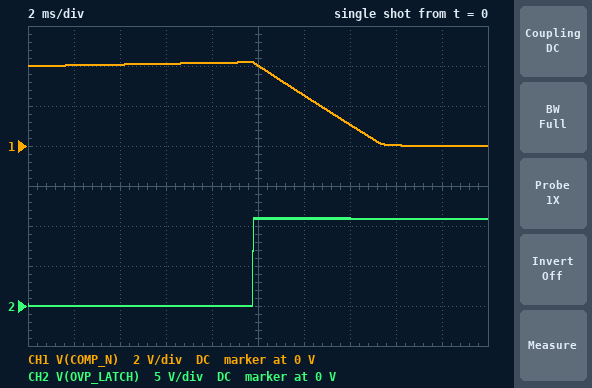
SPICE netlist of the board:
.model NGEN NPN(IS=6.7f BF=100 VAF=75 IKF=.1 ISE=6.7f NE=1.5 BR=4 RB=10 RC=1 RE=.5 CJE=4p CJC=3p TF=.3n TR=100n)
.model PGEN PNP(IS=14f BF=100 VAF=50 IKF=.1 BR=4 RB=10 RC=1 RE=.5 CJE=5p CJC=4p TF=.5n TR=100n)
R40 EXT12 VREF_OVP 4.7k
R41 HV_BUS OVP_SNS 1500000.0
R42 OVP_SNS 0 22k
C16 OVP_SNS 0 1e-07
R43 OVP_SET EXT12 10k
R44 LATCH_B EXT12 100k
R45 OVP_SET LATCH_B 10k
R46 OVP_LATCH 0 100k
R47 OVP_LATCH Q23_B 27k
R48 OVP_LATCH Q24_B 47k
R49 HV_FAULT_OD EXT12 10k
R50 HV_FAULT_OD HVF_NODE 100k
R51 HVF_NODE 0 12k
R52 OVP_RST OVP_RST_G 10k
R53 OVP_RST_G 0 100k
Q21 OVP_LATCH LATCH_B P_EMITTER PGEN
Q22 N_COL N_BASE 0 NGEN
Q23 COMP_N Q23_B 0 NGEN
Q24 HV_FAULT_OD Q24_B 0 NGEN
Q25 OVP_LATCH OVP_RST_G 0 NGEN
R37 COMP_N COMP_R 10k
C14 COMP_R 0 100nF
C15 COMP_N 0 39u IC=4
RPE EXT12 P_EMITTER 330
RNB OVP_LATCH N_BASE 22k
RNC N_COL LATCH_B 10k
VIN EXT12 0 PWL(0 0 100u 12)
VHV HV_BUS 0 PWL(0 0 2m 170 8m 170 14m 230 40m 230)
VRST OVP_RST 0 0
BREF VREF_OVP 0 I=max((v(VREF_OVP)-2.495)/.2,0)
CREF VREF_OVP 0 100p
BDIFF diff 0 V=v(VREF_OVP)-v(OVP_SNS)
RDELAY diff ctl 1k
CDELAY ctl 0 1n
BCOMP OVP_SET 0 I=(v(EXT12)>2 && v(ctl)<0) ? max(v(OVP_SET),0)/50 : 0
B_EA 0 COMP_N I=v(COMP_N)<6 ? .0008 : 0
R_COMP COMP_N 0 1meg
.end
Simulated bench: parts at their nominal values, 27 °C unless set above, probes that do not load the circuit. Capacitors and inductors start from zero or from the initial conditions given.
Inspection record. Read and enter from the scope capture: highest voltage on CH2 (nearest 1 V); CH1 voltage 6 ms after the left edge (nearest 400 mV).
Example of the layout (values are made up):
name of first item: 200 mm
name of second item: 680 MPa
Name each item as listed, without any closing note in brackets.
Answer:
highest voltage on CH2: 11 V
CH1 voltage 6 ms after the left edge: 4.0 V
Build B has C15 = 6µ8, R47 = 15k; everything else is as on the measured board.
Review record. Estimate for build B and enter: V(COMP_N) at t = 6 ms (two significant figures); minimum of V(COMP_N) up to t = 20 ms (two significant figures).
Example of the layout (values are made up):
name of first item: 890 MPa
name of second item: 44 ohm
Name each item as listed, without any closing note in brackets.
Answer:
V(COMP_N) at t = 6 ms: 4.6 V
minimum of V(COMP_N) up to t = 20 ms: 14 mV
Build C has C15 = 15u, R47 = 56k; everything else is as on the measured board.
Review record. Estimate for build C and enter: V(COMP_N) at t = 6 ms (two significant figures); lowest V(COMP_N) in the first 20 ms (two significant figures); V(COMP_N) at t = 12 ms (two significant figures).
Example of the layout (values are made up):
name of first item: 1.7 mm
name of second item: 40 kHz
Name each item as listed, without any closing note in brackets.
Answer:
V(COMP_N) at t = 6 ms: 4.3 V
lowest V(COMP_N) in the first 20 ms: 25 mV
V(COMP_N) at t = 12 ms: 2.2 V
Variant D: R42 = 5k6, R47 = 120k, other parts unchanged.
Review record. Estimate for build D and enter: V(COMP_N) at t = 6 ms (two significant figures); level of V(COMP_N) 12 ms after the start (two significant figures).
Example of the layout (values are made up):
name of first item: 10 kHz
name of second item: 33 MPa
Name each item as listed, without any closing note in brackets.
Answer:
V(COMP_N) at t = 6 ms: 4.1 V
level of V(COMP_N) 12 ms after the start: 4.2 V
